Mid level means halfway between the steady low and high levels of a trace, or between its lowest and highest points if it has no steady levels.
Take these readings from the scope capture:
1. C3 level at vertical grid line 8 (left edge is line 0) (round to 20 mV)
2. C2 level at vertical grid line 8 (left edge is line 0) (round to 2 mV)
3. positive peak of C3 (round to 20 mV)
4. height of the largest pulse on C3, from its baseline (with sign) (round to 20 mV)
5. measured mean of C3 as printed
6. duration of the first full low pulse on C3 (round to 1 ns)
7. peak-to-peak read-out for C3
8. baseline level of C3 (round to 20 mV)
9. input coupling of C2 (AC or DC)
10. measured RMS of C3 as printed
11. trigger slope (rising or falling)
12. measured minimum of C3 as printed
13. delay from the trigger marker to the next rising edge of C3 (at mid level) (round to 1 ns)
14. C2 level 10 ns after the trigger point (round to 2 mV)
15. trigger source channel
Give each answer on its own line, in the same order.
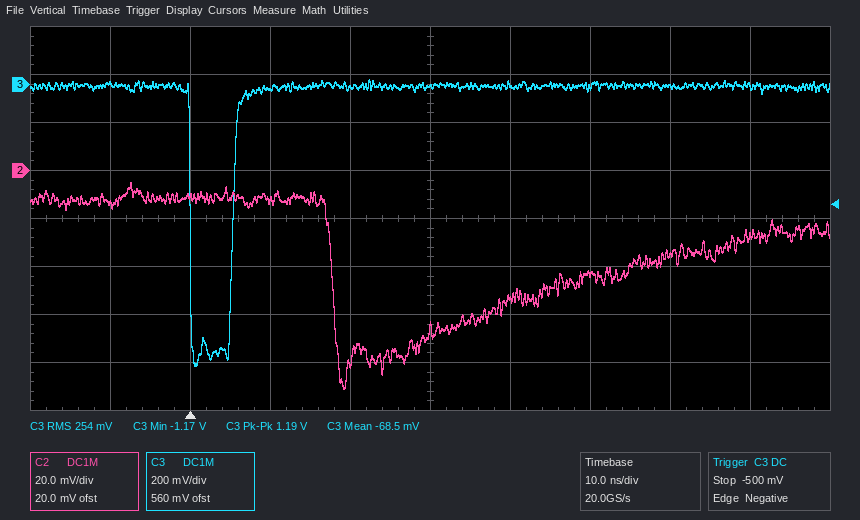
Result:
0 mV
-34 mV
20 mV
-1.16 V
-68.5 mV
5 ns
1.19 V
0 mV
DC
254 mV
falling
-1.17 V
5 ns
-12 mV
C3
